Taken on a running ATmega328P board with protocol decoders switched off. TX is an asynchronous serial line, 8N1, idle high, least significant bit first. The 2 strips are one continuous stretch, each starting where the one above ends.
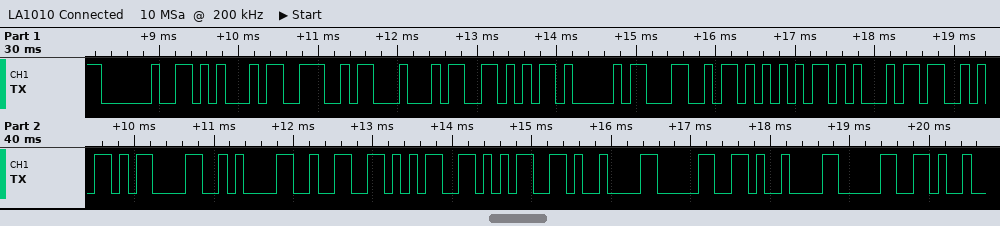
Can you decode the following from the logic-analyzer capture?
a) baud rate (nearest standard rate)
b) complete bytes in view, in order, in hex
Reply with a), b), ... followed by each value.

a) 9600 baud
b) 0x20 0x45 0x4E 0x44 0x56 0x41 0x4C 0x55 0x45 0x53 0x0D 0x0A 0x32 0x35 0x35 0x09 0x30 0x09 0x30
